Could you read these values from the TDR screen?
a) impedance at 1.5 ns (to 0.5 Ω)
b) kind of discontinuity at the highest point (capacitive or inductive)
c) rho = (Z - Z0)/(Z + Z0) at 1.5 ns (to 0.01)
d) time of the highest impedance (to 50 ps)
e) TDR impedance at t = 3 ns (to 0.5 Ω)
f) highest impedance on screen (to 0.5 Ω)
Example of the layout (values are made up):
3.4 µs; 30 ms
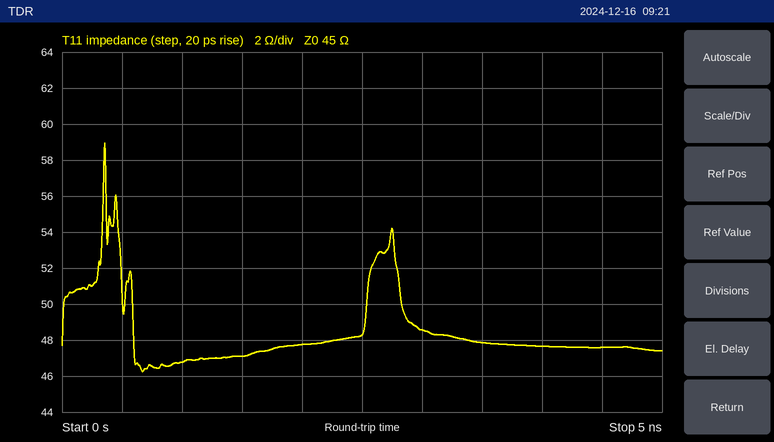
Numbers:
47.0 Ω; inductive; +0.02; 350 ps; 48.5 Ω; 59.0 Ω
